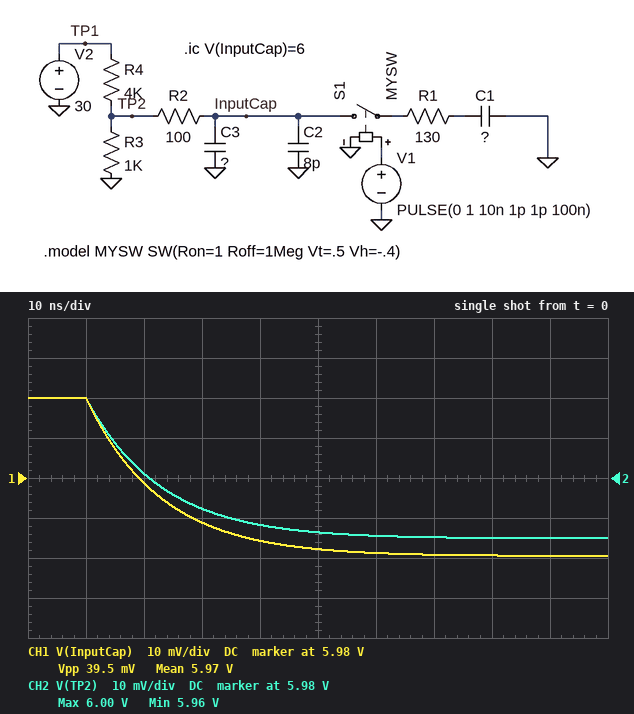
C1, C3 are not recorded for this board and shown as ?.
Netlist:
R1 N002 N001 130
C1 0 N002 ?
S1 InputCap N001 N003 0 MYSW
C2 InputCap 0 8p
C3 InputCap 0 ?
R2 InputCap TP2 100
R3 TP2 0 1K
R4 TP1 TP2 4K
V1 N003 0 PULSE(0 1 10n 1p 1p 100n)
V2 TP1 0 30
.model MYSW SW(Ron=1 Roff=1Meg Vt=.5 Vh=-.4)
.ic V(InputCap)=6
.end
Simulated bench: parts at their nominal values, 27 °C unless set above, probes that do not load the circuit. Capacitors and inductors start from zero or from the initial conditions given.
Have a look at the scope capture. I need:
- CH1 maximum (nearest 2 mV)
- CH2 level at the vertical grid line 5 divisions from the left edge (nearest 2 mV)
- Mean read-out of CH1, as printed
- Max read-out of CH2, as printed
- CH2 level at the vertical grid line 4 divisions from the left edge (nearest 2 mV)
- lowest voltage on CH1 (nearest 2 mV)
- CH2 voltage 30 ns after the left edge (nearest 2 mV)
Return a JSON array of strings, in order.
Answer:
["6.000 V", "5.966 V", "5.97 V", "6.00 V", "5.968 V", "5.960 V", "5.972 V"]
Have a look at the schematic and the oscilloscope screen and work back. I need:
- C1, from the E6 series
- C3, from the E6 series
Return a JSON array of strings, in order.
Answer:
["100 pF", "15 nF"]
